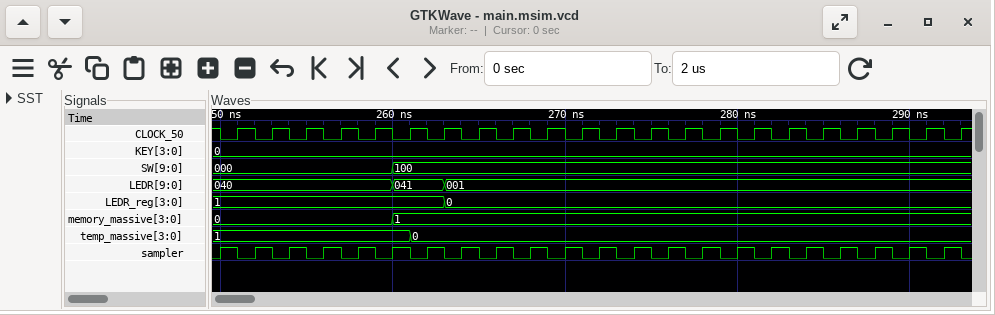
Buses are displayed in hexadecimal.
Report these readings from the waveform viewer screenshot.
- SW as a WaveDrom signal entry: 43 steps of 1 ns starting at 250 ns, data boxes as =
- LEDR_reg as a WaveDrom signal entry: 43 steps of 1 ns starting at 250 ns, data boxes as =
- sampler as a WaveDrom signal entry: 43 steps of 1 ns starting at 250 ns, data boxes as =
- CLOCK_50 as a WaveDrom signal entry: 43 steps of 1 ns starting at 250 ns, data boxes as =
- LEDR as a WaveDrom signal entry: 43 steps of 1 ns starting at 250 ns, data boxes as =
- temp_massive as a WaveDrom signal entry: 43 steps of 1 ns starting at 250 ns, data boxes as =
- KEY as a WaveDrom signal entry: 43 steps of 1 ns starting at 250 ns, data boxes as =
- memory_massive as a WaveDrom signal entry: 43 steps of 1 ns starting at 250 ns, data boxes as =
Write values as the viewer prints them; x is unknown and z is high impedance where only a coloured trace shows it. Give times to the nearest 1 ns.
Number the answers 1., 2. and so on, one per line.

1. {name: 'SW', wave: '=.........=................................', data: '000 100'}
2. {name: 'LEDR_reg', wave: '=............=.............................', data: '1 0'}
3. {name: 'sampler', wave: '1010101010101010101010101010101010101010101'}
4. {name: 'CLOCK_50', wave: '0101010101010101010101010101010101010101010'}
5. {name: 'LEDR', wave: '=.........=..=.............................', data: '040 041 001'}
6. {name: 'temp_massive', wave: '=..........=...............................', data: '1 0'}
7. {name: 'KEY', wave: '=..........................................', data: '0'}
8. {name: 'memory_massive', wave: '=.........=................................', data: '0 1'}
